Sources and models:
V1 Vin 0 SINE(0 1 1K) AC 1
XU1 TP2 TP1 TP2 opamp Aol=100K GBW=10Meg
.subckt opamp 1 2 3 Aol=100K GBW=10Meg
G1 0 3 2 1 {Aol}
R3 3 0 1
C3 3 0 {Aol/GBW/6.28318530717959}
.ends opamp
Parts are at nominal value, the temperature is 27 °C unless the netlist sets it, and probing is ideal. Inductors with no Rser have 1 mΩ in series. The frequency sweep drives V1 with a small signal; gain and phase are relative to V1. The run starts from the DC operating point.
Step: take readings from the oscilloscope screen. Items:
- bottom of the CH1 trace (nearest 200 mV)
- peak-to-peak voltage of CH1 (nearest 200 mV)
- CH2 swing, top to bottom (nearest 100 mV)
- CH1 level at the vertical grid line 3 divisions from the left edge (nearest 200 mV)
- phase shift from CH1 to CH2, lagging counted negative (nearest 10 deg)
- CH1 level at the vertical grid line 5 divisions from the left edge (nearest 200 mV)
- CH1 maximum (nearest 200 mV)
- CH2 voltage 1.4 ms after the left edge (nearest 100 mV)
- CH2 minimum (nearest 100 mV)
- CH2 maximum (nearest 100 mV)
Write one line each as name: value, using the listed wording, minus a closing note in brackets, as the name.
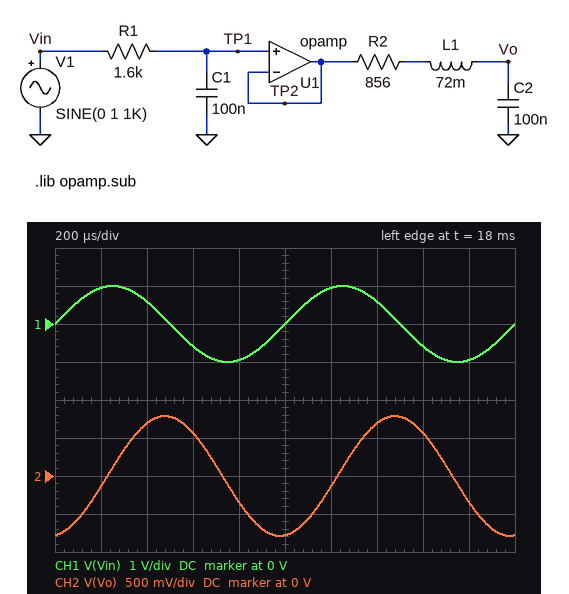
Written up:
bottom of the CH1 trace: -1.0 V
peak-to-peak voltage of CH1: 2.0 V
CH2 swing, top to bottom: 1.6 V
CH1 level at the vertical grid line 3 divisions from the left edge: -600 mV
phase shift from CH1 to CH2, lagging counted negative: -80 deg
CH1 level at the vertical grid line 5 divisions from the left edge: 0 V
CH1 maximum: 1.0 V
CH2 voltage 1.4 ms after the left edge: 700 mV
CH2 minimum: -800 mV
CH2 maximum: 800 mV
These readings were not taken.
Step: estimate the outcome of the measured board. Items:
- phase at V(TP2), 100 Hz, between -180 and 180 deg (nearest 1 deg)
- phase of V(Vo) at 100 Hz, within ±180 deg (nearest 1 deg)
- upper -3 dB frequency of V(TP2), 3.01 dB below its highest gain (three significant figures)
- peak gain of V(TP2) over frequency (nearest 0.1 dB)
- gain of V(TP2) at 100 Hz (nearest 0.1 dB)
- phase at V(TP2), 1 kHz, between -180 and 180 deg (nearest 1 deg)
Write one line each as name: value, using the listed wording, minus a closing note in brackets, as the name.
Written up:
phase at V(TP2), 100 Hz, between -180 and 180 deg: -6 deg
phase of V(Vo) at 100 Hz, within ±180 deg: -9 deg
upper -3 dB frequency of V(TP2), 3.01 dB below its highest gain: 995 Hz
peak gain of V(TP2) over frequency: 0 dB
gain of V(TP2) at 100 Hz: 0 dB
phase at V(TP2), 1 kHz, between -180 and 180 deg: -45 deg
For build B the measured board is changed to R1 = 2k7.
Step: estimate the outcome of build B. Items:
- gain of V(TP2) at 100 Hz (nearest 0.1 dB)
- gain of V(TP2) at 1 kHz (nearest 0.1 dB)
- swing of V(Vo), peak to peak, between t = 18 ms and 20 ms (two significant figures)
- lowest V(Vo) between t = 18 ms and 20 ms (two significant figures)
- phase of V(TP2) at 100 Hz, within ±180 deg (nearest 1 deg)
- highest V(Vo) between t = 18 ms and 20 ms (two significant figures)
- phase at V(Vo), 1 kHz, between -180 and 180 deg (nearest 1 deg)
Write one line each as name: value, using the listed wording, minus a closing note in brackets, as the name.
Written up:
gain of V(TP2) at 100 Hz: -0.1 dB
gain of V(TP2) at 1 kHz: -5.9 dB
swing of V(Vo), peak to peak, between t = 18 ms and 20 ms: 1.1 V
lowest V(Vo) between t = 18 ms and 20 ms: -570 mV
phase of V(TP2) at 100 Hz, within ±180 deg: -10 deg
highest V(Vo) between t = 18 ms and 20 ms: 570 mV
phase at V(Vo), 1 kHz, between -180 and 180 deg: -96 deg
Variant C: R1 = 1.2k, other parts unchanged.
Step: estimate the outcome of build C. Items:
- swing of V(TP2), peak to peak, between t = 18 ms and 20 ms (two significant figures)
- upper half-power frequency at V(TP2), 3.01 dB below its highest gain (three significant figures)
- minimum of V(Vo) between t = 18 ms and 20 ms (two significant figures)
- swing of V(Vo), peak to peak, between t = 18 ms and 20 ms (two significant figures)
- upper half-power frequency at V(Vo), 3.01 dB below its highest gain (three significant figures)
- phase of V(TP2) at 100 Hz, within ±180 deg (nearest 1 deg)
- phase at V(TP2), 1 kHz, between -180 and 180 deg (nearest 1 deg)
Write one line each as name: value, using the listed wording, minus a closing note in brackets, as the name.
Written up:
swing of V(TP2), peak to peak, between t = 18 ms and 20 ms: 1.6 V
upper half-power frequency at V(TP2), 3.01 dB below its highest gain: 1.33 kHz
minimum of V(Vo) between t = 18 ms and 20 ms: -890 mV
swing of V(Vo), peak to peak, between t = 18 ms and 20 ms: 1.8 V
upper half-power frequency at V(Vo), 3.01 dB below its highest gain: 1.60 kHz
phase of V(TP2) at 100 Hz, within ±180 deg: -4 deg
phase at V(TP2), 1 kHz, between -180 and 180 deg: -37 deg
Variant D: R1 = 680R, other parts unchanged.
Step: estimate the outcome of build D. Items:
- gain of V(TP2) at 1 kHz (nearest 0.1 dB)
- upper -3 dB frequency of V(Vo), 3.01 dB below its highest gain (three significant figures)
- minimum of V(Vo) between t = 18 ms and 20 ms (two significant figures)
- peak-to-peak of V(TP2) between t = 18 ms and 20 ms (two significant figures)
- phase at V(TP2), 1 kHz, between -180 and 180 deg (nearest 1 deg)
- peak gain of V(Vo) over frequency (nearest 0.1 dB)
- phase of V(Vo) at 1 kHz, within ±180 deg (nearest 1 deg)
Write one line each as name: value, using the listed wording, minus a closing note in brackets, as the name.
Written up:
gain of V(TP2) at 1 kHz: -0.7 dB
upper -3 dB frequency of V(Vo), 3.01 dB below its highest gain: 1.96 kHz
minimum of V(Vo) between t = 18 ms and 20 ms: -1.0 V
peak-to-peak of V(TP2) between t = 18 ms and 20 ms: 1.8 V
phase at V(TP2), 1 kHz, between -180 and 180 deg: -23 deg
peak gain of V(Vo) over frequency: 0.2 dB
phase of V(Vo) at 1 kHz, within ±180 deg: -60 deg
